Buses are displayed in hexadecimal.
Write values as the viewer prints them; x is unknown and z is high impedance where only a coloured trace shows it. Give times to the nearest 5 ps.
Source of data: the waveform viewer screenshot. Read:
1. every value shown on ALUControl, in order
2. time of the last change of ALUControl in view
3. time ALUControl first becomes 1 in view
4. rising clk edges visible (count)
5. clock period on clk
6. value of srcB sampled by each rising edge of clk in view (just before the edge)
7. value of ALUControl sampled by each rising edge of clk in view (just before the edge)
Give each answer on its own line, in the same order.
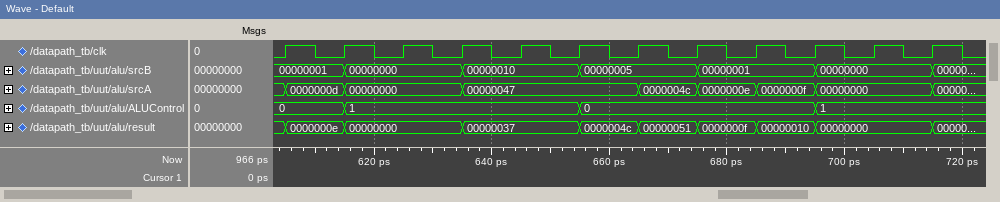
0, 1, 0, 1
695 ps
615 ps
12
10 ps
00000001, 00000001, 00000000, 00000000, 00000010, 00000010, 00000005, 00000005, 00000001, 00000001, 00000000, 00000000
0, 0, 1, 1, 1, 1, 0, 0, 0, 0, 1, 1
